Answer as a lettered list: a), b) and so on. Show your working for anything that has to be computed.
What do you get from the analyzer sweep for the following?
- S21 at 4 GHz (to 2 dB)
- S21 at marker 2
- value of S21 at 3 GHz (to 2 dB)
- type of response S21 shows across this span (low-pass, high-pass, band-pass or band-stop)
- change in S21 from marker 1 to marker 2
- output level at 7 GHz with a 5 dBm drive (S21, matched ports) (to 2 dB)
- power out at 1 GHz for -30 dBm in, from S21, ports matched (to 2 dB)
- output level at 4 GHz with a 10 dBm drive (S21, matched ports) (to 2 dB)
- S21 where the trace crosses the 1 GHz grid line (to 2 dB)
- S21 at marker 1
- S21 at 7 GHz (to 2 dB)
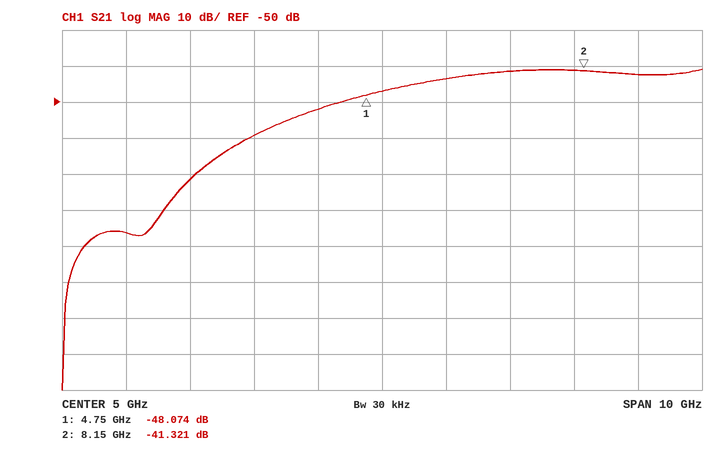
a) -52 dB
b) -41.321 dB
c) -60 dB
d) high-pass
e) -41.321 − (-48.074) = 6.753 dB
f) 5 dBm + (-42 dB) = -36 dBm
g) -30 dBm + (-86 dB) = -116 dBm
h) 10 dBm + (-52 dB) = -42 dBm
i) -86 dB
j) -48.074 dB
k) -42 dB
